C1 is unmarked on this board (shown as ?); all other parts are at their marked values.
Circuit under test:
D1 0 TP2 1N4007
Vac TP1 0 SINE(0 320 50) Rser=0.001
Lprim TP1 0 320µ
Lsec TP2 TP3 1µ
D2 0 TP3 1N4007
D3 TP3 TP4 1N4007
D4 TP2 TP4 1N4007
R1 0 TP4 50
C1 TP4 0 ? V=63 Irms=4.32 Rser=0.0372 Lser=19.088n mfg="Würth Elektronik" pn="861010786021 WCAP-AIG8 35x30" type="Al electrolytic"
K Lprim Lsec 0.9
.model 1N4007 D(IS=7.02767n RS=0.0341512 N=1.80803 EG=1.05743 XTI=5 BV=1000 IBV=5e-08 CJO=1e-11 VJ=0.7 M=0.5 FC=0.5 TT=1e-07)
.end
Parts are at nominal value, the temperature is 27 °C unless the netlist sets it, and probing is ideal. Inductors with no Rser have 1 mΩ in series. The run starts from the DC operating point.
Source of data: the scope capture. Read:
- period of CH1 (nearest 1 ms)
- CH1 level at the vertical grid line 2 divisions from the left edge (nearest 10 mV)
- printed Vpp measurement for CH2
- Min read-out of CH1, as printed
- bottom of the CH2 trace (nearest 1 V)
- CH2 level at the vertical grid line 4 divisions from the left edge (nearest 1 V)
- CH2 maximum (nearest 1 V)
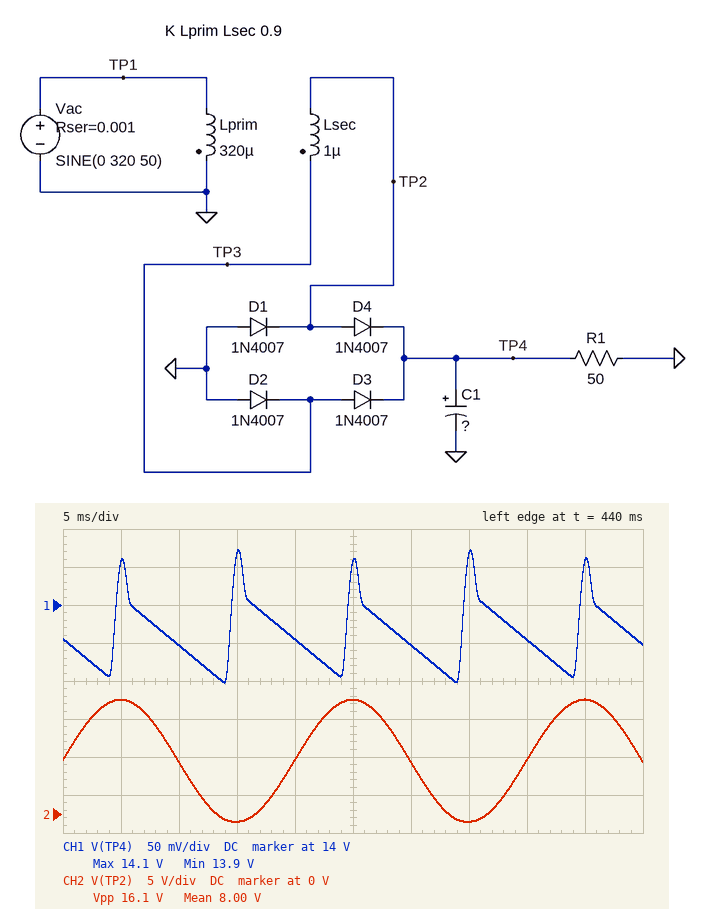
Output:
10 ms
13.95 V
16.1 V
13.9 V
-1 V
7 V
15 V
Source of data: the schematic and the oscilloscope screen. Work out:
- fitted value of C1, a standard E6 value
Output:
22 mF
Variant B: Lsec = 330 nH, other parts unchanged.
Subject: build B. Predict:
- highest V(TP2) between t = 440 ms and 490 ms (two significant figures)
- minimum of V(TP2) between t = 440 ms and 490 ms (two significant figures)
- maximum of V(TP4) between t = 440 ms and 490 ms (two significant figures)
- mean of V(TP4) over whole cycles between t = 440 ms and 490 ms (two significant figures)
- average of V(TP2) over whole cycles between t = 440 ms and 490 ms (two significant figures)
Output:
8.3 V
-940 mV
7.4 V
7.3 V
3.7 V
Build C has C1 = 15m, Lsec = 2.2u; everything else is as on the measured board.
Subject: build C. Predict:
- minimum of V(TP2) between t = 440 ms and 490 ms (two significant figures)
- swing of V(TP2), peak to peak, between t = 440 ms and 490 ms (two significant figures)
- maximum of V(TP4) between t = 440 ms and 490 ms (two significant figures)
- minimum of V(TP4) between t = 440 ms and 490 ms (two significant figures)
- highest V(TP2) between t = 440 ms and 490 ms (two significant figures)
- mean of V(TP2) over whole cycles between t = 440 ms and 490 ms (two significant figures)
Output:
-1.1 V
24 V
22 V
21 V
23 V
11 V
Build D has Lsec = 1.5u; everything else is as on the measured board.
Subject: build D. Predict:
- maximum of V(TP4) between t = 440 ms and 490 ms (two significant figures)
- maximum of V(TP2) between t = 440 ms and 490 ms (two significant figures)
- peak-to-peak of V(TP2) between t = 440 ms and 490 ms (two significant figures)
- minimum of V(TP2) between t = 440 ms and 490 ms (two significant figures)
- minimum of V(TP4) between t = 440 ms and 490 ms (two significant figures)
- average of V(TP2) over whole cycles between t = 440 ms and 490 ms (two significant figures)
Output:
18 V
19 V
20 V
-1.1 V
17 V
8.7 V
